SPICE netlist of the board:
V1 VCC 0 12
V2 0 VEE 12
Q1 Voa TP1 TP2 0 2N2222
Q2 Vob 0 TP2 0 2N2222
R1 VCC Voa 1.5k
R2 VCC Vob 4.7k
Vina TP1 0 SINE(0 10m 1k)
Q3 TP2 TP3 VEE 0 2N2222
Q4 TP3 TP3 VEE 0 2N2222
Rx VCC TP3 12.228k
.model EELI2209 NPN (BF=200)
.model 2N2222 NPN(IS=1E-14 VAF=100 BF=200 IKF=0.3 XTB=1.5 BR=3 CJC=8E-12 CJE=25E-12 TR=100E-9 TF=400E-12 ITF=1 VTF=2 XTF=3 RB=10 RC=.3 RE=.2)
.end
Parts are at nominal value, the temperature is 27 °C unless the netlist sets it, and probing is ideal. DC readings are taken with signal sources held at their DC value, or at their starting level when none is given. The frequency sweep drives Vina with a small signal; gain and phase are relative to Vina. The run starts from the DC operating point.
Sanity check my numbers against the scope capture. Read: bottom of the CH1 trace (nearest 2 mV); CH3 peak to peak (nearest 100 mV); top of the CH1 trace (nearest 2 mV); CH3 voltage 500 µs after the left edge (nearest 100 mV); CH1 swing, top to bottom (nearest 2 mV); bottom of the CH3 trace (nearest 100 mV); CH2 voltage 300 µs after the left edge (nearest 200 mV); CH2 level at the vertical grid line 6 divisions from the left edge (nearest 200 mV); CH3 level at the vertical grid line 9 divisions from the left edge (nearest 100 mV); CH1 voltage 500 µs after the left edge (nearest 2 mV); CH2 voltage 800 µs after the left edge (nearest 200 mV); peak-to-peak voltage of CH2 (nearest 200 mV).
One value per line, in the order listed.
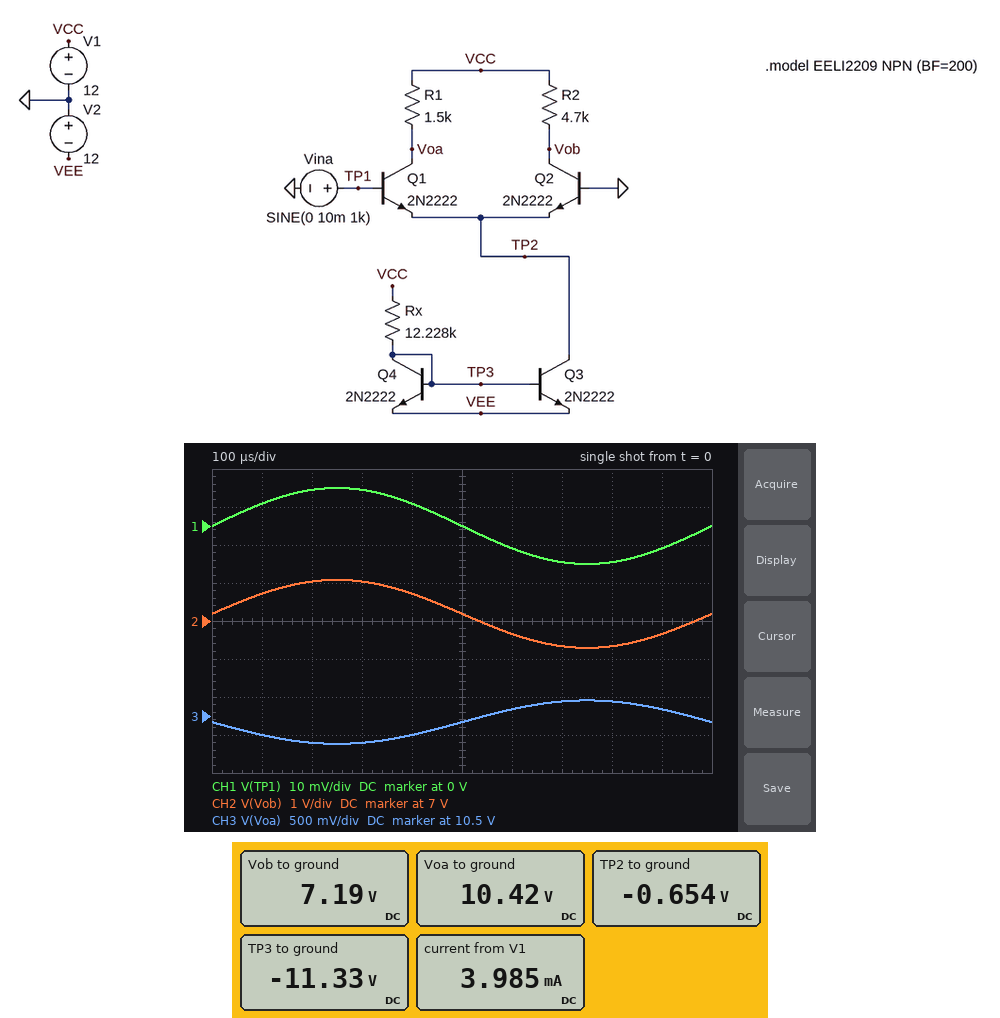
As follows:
-10 mV
600 mV
10 mV
10.4 V
20 mV
10.1 V
8.0 V
6.6 V
10.6 V
0 V
6.4 V
1.8 V
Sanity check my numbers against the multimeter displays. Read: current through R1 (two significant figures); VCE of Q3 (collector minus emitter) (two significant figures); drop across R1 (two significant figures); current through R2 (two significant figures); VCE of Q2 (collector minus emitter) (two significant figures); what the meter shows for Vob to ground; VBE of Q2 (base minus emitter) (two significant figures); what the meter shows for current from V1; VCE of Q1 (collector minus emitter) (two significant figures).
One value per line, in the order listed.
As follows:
1.1 mA
11 V
1.6 V
1.0 mA
7.8 V
7.19 V
650 mV
3.985 mA
11 V
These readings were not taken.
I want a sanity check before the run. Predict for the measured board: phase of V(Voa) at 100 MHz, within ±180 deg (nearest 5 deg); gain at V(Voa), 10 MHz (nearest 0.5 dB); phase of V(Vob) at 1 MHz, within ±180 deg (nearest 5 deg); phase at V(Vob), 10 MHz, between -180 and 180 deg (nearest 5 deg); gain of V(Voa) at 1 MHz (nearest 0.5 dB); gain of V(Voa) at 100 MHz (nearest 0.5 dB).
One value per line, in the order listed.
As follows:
85 deg
28.0 dB
-10 deg
-55 deg
29.0 dB
16.5 dB
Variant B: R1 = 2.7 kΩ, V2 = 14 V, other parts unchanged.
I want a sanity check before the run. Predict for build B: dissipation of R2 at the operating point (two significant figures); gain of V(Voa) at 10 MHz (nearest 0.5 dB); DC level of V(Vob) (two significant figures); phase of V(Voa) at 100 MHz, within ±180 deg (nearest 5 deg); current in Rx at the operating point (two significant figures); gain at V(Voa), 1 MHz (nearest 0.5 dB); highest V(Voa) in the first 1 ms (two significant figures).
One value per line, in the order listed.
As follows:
6.1 mW
32.5 dB
6.7 V
80 deg
2.1 mA
35.0 dB
9.4 V
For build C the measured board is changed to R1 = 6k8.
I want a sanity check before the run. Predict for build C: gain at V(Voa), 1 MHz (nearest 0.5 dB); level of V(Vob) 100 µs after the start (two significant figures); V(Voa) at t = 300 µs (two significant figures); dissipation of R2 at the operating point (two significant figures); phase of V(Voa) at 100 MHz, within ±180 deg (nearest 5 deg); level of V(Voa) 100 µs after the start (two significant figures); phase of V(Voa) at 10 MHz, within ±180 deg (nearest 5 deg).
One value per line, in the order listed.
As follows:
42.0 dB
7.6 V
3.8 V
5.2 mW
70 deg
4.3 V
110 deg
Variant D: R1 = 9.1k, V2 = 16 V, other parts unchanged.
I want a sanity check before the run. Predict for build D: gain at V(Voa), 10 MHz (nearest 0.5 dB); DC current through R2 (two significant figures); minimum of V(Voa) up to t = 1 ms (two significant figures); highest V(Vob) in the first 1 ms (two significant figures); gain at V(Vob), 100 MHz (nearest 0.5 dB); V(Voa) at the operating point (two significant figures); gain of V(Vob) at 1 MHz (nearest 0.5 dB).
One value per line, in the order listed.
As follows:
32.5 dB
1.3 mA
-580 mV
6.8 V
15.5 dB
820 mV
40.0 dB
